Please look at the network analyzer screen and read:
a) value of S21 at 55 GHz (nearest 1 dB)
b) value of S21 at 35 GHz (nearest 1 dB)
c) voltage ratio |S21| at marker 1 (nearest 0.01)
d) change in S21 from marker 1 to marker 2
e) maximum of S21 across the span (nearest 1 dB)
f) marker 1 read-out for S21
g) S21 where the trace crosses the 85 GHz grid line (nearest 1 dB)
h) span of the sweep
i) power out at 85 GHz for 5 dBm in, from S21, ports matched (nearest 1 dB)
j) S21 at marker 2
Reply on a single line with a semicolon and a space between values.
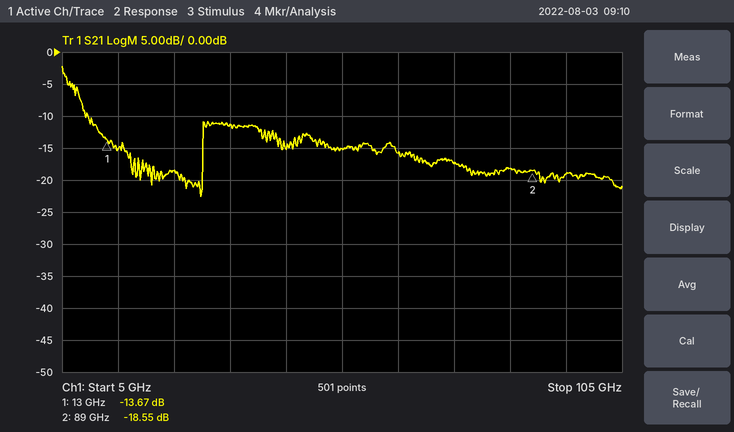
-15 dB; -11 dB; 0.21; -4.88 dB; -2 dB; -13.67 dB; -18 dB; 100 GHz; -13 dBm; -18.55 dB
